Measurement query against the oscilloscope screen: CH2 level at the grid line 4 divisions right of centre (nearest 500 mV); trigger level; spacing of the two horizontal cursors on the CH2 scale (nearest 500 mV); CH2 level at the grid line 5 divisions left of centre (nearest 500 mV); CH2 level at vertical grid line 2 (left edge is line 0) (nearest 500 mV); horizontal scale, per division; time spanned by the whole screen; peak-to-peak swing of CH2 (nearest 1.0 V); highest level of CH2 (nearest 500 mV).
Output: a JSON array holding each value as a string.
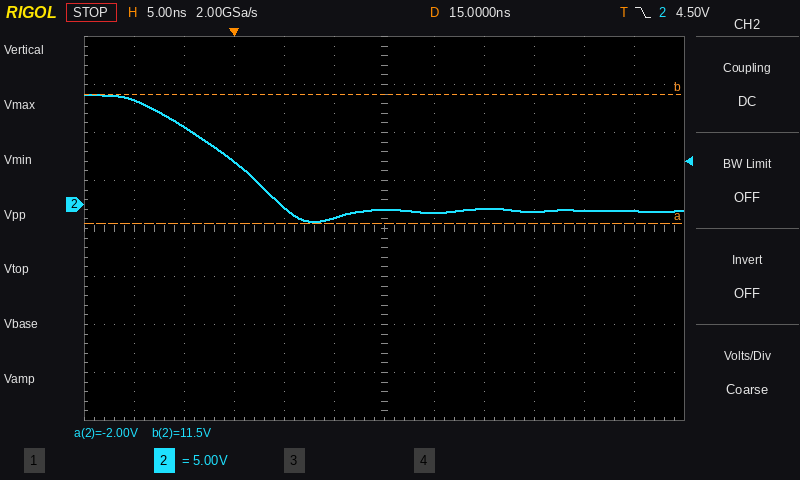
["-500 mV", "4.50 V", "13.5 V", "11.0 V", "8.0 V", "5 ns", "60 ns", "13.0 V", "11.5 V"]
